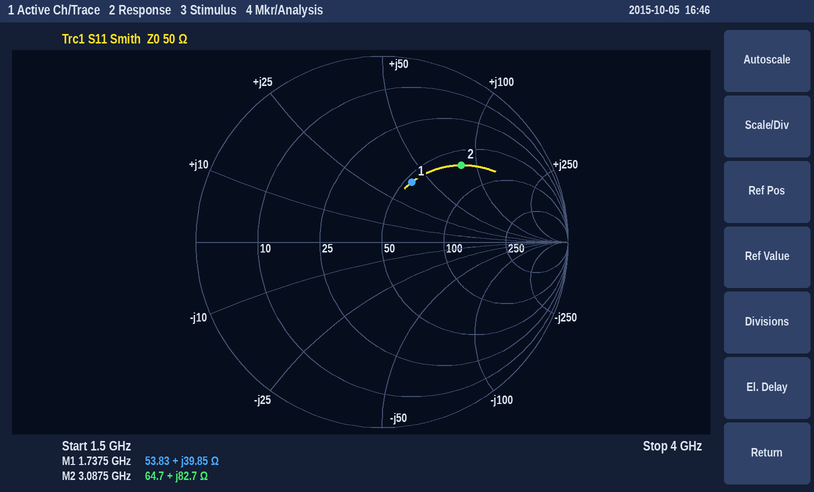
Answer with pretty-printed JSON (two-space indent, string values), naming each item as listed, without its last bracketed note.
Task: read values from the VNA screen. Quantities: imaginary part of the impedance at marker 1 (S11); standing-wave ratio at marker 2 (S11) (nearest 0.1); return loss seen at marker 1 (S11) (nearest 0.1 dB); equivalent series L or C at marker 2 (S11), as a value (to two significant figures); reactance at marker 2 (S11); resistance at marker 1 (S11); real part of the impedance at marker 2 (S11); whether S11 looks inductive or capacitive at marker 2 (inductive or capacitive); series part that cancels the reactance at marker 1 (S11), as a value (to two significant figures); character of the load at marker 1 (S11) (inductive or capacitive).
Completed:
{
  "imaginary part of the impedance at marker 1": "+39.85 Ω",
  "standing-wave ratio at marker 2 (S11)": "3.9",
  "return loss seen at marker 1 (S11)": "8.9 dB",
  "equivalent series L or C at marker 2 (S11), as a value": "4.3 nH",
  "reactance at marker 2": "+82.7 Ω",
  "resistance at marker 1": "53.83 Ω",
  "real part of the impedance at marker 2": "64.7 Ω",
  "whether S11 looks inductive or capacitive at marker 2": "inductive",
  "series part that cancels the reactance at marker 1 (S11), as a value": "2.3 pF",
  "character of the load at marker 1 (S11)": "inductive"
}
